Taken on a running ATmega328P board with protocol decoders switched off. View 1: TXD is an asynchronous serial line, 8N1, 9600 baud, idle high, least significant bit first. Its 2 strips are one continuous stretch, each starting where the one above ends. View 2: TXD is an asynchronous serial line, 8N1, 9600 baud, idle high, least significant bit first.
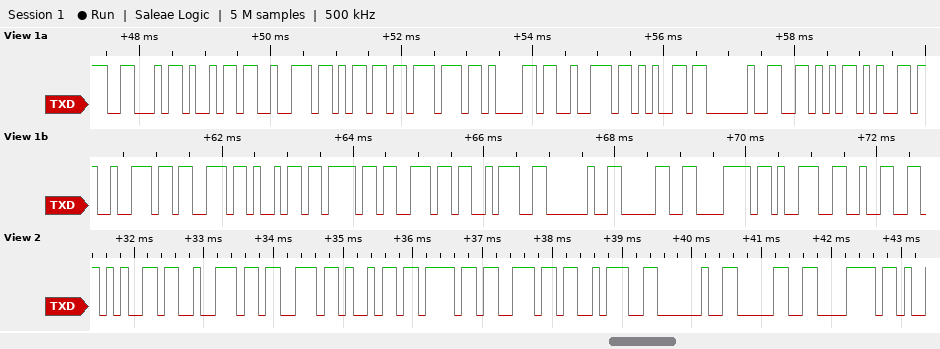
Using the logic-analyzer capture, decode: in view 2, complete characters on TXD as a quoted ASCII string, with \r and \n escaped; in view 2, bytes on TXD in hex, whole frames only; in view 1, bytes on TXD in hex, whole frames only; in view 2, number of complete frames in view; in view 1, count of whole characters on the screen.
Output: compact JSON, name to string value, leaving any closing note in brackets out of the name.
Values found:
{"in view 2, complete characters on TXD as a quoted ASCII string, with \\r and \\n escaped": "\"ersion: 0x\"", "in view 2, bytes on TXD in hex, whole frames only": "65 72 73 69 6F 6E 3A 20 30 78", "in view 1, bytes on TXD in hex, whole frames only": "0x46 0x69 0x72 0x6D 0x77 0x61 0x72 0x65 0x20 0x56 0x65 0x72 0x73 0x69 0x6F 0x6E 0x3A 0x20 0x30 0x78 0x39 0x32", "in view 2, number of complete frames in view": "10", "in view 1, count of whole characters on the screen": "22"}
